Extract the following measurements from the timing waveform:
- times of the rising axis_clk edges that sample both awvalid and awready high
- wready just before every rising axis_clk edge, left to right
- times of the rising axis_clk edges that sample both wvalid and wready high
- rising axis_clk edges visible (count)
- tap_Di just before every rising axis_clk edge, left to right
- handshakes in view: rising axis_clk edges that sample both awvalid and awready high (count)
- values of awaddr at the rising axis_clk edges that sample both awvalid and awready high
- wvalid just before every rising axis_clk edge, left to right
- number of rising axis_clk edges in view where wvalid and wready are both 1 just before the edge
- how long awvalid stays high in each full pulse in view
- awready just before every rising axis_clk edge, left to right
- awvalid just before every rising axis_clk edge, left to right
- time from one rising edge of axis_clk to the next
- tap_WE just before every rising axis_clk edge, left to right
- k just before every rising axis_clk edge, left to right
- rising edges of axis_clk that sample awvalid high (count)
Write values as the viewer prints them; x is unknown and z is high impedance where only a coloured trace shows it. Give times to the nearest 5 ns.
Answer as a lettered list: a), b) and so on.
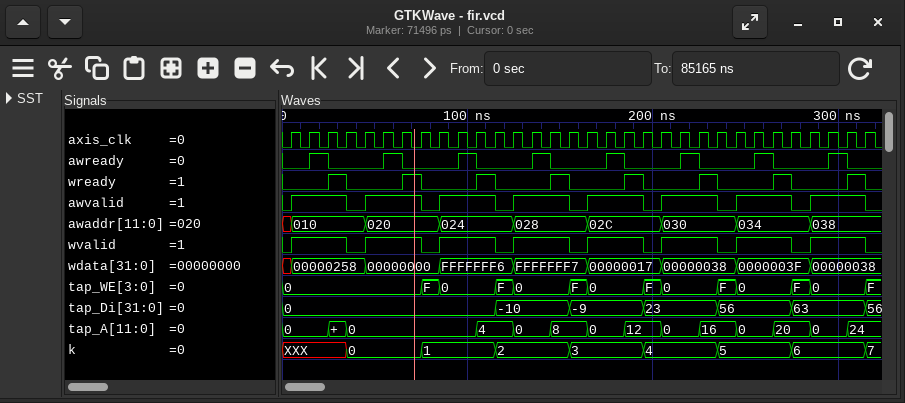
a) 25 ns, 65 ns, 105 ns, 145 ns, 185 ns, 225 ns, 265 ns, 305 ns
b) 0 0 0 1 0 0 0 1 0 0 0 1 0 0 0 1 0 0 0 1 0 0 0 1 0 0 0 1 0 0 0 1
c) 35 ns, 75 ns, 115 ns, 155 ns, 195 ns, 235 ns, 275 ns, 315 ns
d) 32
e) 0, 0, 0, 0, 0, 0, 0, 0, 0, 0, 0, 0, -10, -10, -10, -10, -9, -9, -9, -9, 23, 23, 23, 23, 56, 56, 56, 56, 63, 63, 63, 63
f) 8
g) 010, 020, 024, 028, 02C, 030, 034, 038
h) 0 1 1 1 0 1 1 1 0 1 1 1 0 1 1 1 0 1 1 1 0 1 1 1 0 1 1 1 0 1 1 1
i) 8
j) 30 ns, 30 ns, 30 ns, 30 ns, 30 ns, 30 ns, 30 ns, 30 ns
k) 0 0 1 0 0 0 1 0 0 0 1 0 0 0 1 0 0 0 1 0 0 0 1 0 0 0 1 0 0 0 1 0
l) 0 1 1 1 0 1 1 1 0 1 1 1 0 1 1 1 0 1 1 1 0 1 1 1 0 1 1 1 0 1 1 1
m) 10 ns
n) 0, 0, 0, 0, 0, 0, 0, 0, F, 0, 0, 0, F, 0, 0, 0, F, 0, 0, 0, F, 0, 0, 0, F, 0, 0, 0, F, 0, 0, 0
o) XXX, XXX, XXX, XXX, 0, 0, 0, 0, 1, 1, 1, 1, 2, 2, 2, 2, 3, 3, 3, 3, 4, 4, 4, 4, 5, 5, 5, 5, 6, 6, 6, 6
p) 24
